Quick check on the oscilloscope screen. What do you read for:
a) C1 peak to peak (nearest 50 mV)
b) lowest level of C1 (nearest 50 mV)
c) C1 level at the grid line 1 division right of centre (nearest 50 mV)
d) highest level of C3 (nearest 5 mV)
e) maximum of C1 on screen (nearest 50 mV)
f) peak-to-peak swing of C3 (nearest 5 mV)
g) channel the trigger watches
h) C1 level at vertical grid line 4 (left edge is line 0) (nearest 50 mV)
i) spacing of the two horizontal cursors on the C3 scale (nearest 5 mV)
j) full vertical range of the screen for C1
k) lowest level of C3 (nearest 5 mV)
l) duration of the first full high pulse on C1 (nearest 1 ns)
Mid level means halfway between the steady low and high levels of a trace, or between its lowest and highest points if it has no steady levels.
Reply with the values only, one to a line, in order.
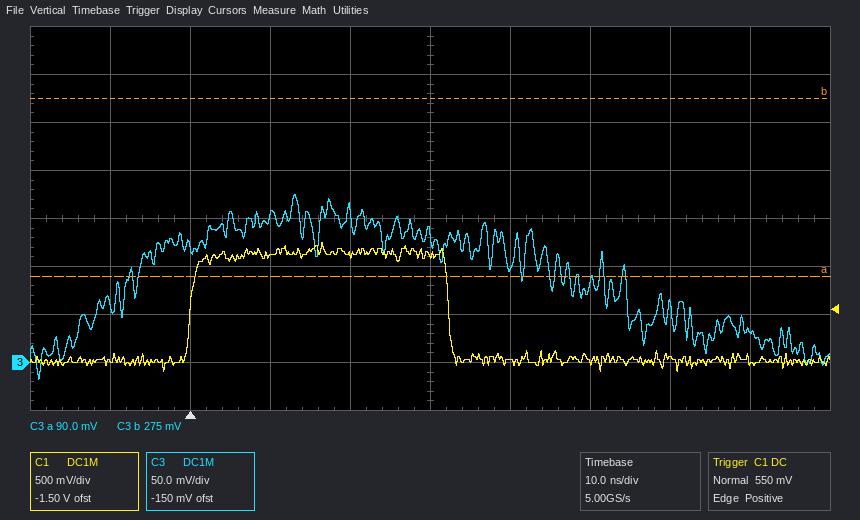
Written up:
1.35 V
-100 mV
0 mV
175 mV
1.25 V
195 mV
C1
1.10 V
185 mV
4 V
-20 mV
32 ns
